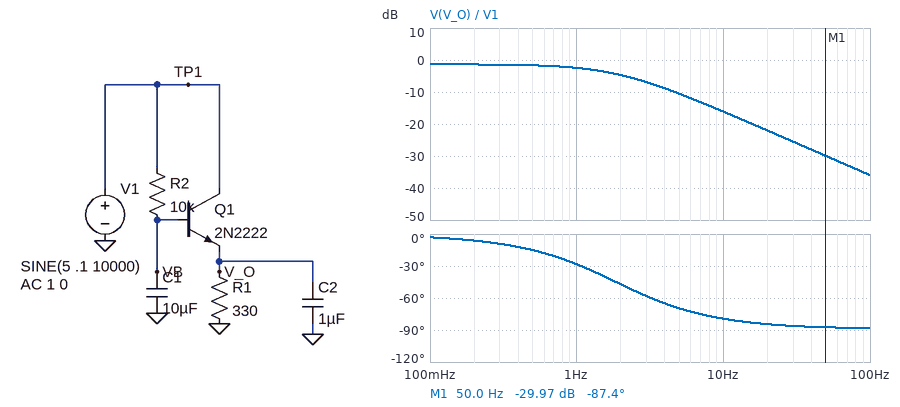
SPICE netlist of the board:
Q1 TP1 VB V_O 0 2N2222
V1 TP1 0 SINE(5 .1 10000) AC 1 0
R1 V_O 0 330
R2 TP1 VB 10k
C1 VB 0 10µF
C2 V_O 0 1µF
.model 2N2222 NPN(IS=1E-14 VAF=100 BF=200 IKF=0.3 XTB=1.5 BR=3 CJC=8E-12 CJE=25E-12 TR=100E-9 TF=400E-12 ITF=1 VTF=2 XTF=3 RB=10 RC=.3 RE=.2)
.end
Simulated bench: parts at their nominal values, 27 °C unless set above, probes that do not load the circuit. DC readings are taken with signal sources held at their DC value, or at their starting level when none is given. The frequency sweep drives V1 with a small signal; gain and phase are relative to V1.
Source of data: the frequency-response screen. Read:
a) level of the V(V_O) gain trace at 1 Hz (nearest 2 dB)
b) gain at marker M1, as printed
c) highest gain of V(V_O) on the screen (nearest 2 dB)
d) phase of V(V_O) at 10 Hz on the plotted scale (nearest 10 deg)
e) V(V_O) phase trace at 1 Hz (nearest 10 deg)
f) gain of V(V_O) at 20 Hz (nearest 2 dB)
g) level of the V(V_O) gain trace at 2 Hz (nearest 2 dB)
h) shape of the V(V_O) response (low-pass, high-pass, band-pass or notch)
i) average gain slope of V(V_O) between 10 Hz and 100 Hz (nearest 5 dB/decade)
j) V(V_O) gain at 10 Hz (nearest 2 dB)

-2 dB
-29.97 dB
-2 dB
-80 deg
-30 deg
-22 dB
-4 dB
low-pass
-20 dB/decade
-16 dB
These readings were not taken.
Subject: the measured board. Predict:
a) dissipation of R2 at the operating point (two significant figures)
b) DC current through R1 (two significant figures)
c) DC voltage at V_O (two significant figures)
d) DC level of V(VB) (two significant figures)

33 µW
11 mA
3.7 V
4.4 V
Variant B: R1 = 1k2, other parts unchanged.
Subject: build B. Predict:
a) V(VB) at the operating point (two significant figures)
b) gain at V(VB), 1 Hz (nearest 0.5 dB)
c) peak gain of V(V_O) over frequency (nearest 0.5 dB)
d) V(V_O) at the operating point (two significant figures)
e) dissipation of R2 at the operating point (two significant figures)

4.8 V
-1.5 dB
-0.5 dB
4.1 V
3.0 µW
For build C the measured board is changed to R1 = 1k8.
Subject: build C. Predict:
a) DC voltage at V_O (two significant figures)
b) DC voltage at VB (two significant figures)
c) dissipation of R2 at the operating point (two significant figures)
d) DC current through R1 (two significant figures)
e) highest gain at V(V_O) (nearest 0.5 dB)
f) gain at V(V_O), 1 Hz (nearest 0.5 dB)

4.2 V
4.9 V
1.4 µW
2.3 mA
-0.5 dB
-1.5 dB
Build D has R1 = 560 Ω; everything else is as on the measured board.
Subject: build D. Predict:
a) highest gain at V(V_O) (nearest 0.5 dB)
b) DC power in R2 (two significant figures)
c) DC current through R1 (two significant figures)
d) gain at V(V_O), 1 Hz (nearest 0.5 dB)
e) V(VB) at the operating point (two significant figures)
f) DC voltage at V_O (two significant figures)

-1.0 dB
13 µW
7.0 mA
-2.0 dB
4.6 V
3.9 V
